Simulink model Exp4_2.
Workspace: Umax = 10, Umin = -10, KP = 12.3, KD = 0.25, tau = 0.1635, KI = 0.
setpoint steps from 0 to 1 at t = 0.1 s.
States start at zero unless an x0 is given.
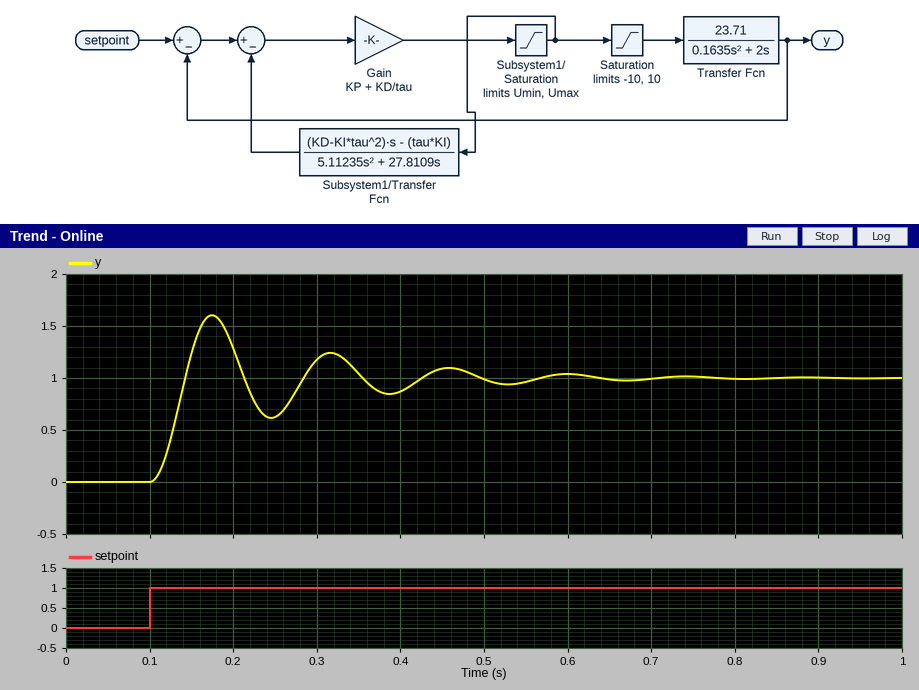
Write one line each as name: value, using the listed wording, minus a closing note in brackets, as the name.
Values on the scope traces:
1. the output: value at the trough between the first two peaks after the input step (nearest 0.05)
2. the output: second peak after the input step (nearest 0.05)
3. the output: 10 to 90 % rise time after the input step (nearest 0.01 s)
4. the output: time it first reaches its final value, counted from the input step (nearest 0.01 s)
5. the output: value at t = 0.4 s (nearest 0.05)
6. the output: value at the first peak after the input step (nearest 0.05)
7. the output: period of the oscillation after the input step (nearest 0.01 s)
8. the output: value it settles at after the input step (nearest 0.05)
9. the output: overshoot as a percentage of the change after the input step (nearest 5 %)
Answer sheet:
the output: value at the trough between the first two peaks after the input step: 0.60
the output: second peak after the input step: 1.25
the output: 10 to 90 % rise time after the input step: 0.03 s
the output: time it first reaches its final value, counted from the input step: 0.04 s
the output: value at t = 0.4 s: 0.85
the output: value at the first peak after the input step: 1.60
the output: period of the oscillation after the input step: 0.14 s
the output: value it settles at after the input step: 1.00
the output: overshoot as a percentage of the change after the input step: 60 %
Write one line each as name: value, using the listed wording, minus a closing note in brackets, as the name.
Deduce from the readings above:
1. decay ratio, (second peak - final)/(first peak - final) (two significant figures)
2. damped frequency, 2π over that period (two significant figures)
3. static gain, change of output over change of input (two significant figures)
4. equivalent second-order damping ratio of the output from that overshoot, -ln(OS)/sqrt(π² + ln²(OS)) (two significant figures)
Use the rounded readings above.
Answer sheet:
decay ratio, (second peak - final)/(first peak - final): 0.42
damped frequency, 2π over that period: 45 rad/s
static gain, change of output over change of input: 1.0
equivalent second-order damping ratio of the output from that overshoot, -ln(OS)/sqrt(π² + ln²(OS)): 0.16
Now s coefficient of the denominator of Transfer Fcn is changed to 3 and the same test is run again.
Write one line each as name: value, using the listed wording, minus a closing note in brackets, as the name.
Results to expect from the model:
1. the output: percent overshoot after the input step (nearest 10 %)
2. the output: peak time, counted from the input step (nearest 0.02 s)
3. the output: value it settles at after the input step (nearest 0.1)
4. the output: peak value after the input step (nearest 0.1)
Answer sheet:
the output: percent overshoot after the input step: 50 %
the output: peak time, counted from the input step: 0.08 s
the output: value it settles at after the input step: 1.0
the output: peak value after the input step: 1.5
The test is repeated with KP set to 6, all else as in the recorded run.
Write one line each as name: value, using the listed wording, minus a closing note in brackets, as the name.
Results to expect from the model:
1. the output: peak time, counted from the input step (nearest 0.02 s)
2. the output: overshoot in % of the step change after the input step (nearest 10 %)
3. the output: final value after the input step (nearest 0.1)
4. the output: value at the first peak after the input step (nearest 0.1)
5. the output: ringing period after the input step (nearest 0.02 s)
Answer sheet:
the output: peak time, counted from the input step: 0.10 s
the output: overshoot in % of the step change after the input step: 50 %
the output: final value after the input step: 1.0
the output: value at the first peak after the input step: 1.5
the output: ringing period after the input step: 0.20 s
